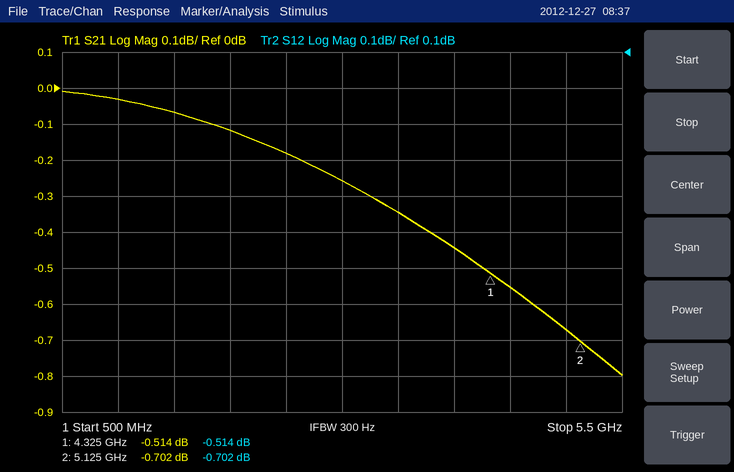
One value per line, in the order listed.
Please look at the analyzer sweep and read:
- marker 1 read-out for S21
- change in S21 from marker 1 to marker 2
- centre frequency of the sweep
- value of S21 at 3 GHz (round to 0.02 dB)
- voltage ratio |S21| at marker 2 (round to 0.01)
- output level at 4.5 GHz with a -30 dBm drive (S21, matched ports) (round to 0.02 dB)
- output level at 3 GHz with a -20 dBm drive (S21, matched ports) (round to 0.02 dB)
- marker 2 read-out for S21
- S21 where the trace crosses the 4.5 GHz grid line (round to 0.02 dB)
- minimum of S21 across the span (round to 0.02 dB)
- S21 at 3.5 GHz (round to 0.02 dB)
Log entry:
-0.514 dB
-0.188 dB
3 GHz
-0.26 dB
0.92
-30.56 dBm
-20.26 dBm
-0.702 dB
-0.56 dB
-0.80 dB
-0.34 dB
